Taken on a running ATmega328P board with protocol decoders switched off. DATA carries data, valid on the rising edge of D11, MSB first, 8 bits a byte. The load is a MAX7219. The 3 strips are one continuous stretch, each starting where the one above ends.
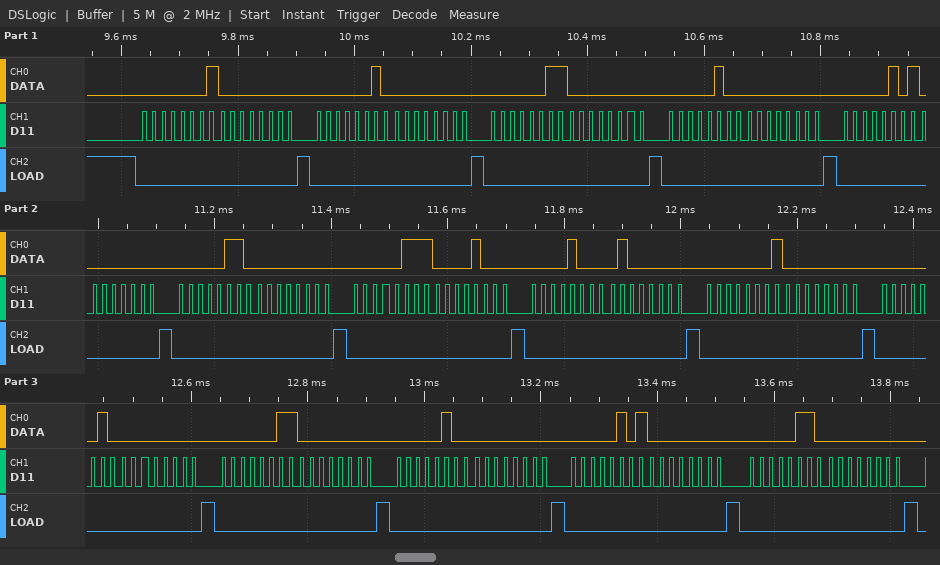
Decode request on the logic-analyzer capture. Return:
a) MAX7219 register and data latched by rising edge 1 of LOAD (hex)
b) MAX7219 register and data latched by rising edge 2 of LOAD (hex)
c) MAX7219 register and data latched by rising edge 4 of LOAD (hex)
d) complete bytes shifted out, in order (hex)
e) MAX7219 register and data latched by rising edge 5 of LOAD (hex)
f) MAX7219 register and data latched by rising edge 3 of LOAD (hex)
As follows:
register 0x1, data 0x00
register 0x2, data 0x00
register 0x4, data 0x00
0x01 0x00 0x02 0x00 0x03 0x00 0x04 0x00 0x05 0x00 0x06 0x00 0x07 0x08 0x08 0x40 0x01 0x00 0x02 0x00 0x03 0x00 0x04 0x00 0x05 0x00 0x06 0x00
register 0x5, data 0x00
register 0x3, data 0x00
